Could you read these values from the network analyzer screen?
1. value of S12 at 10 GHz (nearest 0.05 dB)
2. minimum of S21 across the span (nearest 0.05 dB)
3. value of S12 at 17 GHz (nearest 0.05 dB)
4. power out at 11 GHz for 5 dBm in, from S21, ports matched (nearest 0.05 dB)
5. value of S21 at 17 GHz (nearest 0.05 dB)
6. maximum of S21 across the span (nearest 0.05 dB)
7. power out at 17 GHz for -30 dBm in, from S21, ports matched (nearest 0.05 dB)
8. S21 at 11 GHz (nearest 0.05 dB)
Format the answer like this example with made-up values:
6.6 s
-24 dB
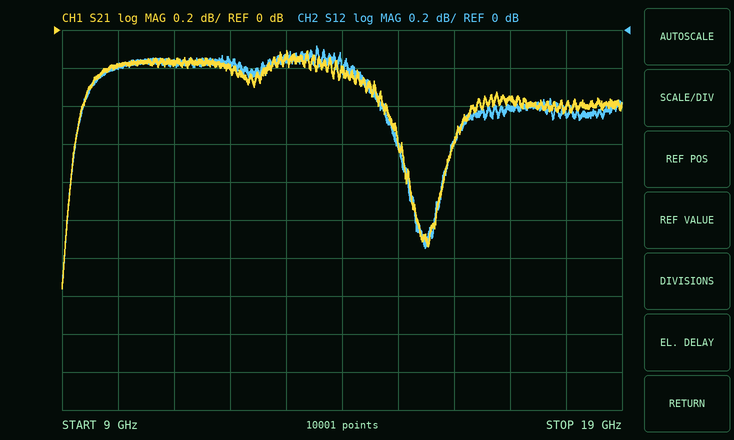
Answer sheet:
-0.20 dB
-1.35 dB
-0.40 dB
4.85 dBm
-0.35 dB
-0.10 dB
-30.35 dBm
-0.15 dB
